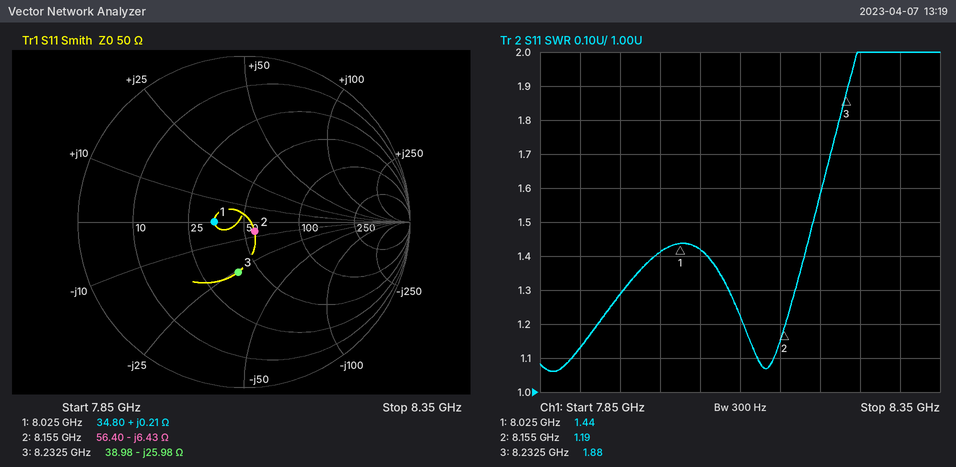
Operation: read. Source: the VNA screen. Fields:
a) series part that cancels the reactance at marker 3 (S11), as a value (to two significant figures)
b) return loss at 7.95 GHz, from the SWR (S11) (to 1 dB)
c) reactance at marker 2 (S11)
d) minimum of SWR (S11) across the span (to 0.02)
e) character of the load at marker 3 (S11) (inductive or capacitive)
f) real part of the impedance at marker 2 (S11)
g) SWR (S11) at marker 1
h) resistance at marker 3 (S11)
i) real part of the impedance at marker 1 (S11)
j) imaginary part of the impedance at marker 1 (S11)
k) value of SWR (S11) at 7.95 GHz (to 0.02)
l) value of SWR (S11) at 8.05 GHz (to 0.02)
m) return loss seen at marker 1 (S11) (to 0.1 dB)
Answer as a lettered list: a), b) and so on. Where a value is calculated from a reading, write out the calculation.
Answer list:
a) L = 25.98 Ω/(2π × 8.2325 GHz) ≈ 502 pH, so 500 pH to two significant figures
b) −20 log10((1.28 − 1)/(1.28 + 1)) ≈ 18 dB
c) -6.43 Ω
d) 1.06
e) capacitive
f) 56.40 Ω
g) 1.44
h) 38.98 Ω
i) 34.80 Ω
j) +0.21 Ω
k) 1.28
l) 1.42
m) 14.9 dB
